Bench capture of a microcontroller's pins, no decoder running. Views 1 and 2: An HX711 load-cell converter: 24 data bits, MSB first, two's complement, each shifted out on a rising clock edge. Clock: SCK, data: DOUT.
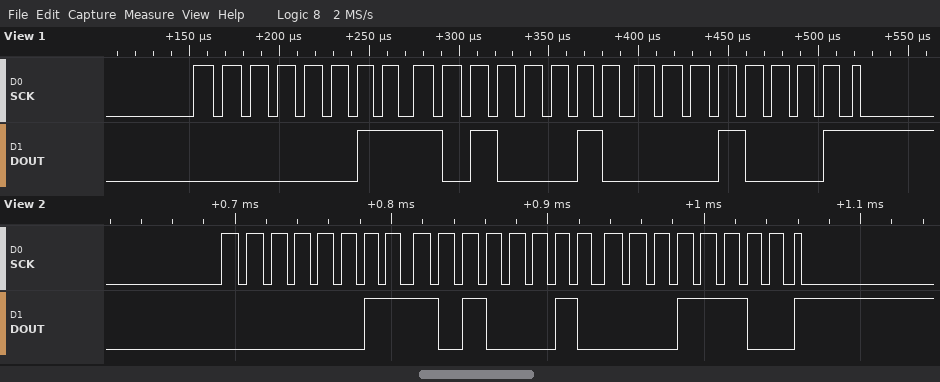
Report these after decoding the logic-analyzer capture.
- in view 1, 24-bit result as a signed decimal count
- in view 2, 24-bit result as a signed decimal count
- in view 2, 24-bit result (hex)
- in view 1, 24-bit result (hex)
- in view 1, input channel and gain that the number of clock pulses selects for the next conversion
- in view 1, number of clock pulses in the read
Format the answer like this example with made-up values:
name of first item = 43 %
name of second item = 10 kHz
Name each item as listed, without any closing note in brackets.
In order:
in view 1, 24-bit result as a signed decimal count = 238097
in view 2, 24-bit result as a signed decimal count = 238108
in view 2, 24-bit result = 0x03A21C
in view 1, 24-bit result = 0x03A211
in view 1, input channel and gain that the number of clock pulses selects for the next conversion = channel A, gain 128
in view 1, number of clock pulses in the read = 25
